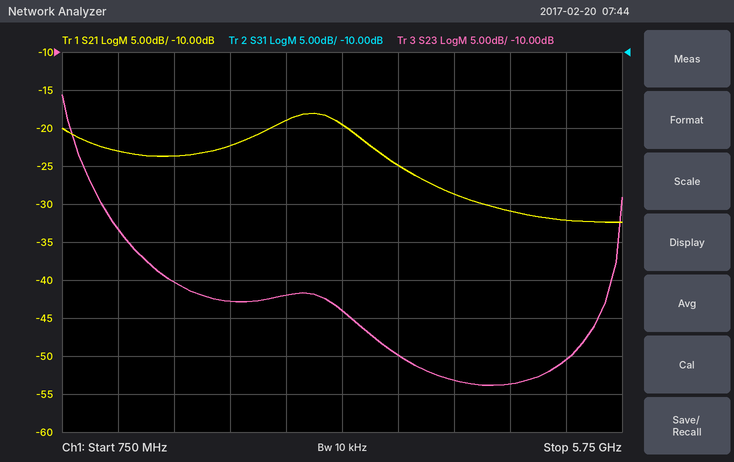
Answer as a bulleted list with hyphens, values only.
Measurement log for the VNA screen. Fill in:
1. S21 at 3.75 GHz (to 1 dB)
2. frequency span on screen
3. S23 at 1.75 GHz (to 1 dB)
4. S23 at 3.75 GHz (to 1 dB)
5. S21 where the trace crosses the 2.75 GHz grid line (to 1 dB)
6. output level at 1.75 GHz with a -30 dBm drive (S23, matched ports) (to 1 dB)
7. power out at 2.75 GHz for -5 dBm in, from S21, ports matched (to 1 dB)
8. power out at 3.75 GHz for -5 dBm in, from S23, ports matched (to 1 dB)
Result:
- -25 dB
- 5 GHz
- -40 dB
- -50 dB
- -19 dB
- -70 dBm
- -24 dBm
- -55 dBm
